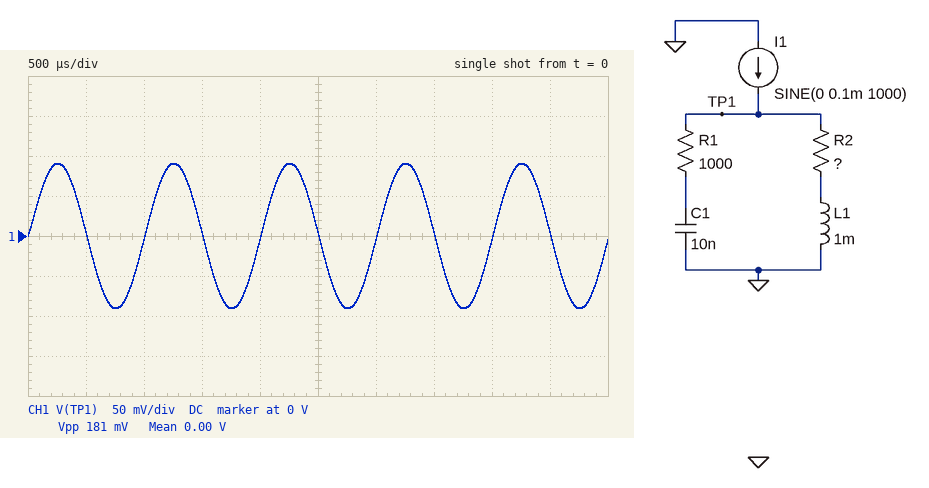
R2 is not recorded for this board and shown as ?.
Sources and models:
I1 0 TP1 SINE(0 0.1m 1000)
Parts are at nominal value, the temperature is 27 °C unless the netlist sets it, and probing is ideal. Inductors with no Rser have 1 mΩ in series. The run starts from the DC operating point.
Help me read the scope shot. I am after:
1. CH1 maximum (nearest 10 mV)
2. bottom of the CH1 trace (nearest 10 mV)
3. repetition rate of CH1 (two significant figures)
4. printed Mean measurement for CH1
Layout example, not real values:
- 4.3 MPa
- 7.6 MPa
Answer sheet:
- 90 mV
- -90 mV
- 1.0 kHz
- 0.00 V
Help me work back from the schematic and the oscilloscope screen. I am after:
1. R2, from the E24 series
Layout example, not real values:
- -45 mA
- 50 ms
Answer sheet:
- 910 Ω
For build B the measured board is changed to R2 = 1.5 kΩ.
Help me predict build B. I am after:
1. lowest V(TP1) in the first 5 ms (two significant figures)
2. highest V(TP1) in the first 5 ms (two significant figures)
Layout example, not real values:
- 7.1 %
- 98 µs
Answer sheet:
- -150 mV
- 150 mV
